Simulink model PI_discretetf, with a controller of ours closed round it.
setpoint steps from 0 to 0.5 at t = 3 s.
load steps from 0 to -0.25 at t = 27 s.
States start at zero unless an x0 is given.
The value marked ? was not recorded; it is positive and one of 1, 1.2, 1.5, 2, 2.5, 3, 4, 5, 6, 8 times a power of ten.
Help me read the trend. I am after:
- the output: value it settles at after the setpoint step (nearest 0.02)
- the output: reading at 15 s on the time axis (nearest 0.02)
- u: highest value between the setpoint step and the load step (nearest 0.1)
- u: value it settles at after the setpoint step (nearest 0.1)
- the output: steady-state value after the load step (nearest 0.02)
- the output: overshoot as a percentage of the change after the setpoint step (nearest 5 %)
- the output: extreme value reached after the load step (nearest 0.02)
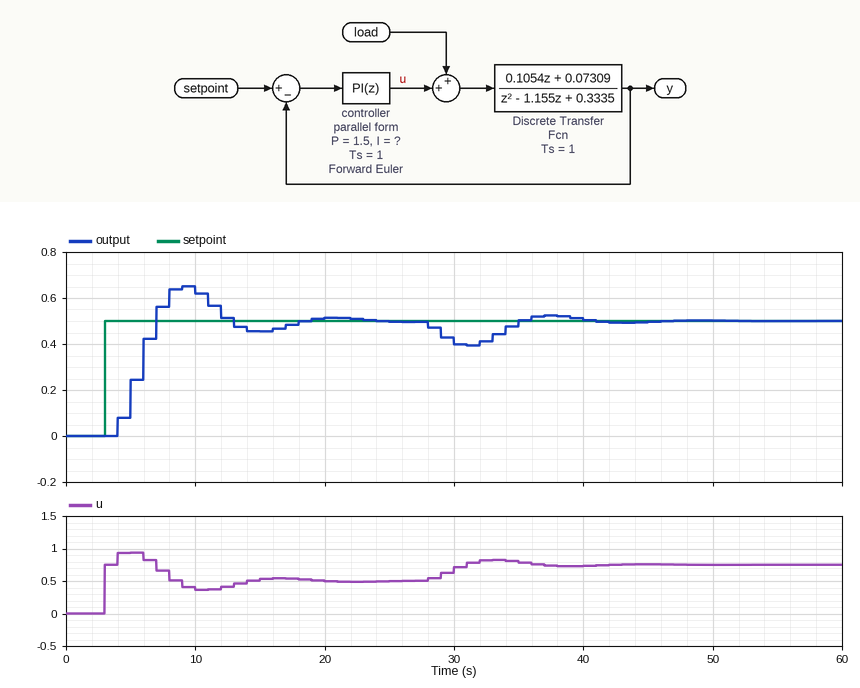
0.50
0.46
0.9
0.5
0.50
30 %
0.40
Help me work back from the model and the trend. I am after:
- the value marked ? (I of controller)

0.6
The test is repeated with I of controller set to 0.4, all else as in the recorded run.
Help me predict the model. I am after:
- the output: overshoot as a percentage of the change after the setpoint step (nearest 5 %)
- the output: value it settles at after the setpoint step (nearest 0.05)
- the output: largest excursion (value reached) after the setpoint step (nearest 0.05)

10 %
0.50
0.55
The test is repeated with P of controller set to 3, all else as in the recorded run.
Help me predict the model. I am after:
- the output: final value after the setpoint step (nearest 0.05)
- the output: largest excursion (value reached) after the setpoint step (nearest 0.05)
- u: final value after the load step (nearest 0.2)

0.50
0.65
0.8
